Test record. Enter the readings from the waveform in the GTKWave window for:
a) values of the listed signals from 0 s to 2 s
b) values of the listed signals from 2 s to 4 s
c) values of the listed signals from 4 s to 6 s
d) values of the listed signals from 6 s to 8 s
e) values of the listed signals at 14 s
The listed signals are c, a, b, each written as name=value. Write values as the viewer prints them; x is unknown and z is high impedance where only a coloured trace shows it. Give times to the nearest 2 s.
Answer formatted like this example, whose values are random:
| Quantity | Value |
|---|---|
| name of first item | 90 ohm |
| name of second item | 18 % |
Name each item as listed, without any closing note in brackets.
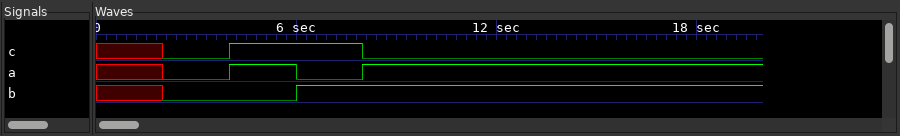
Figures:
| Quantity | Value |
|---|---|
| values of the listed signals from 0 s to 2 s | c=x, a=x, b=x |
| values of the listed signals from 2 s to 4 s | c=0, a=0, b=0 |
| values of the listed signals from 4 s to 6 s | c=1, a=1, b=0 |
| values of the listed signals from 6 s to 8 s | c=1, a=0, b=1 |
| values of the listed signals at 14 s | c=0, a=1, b=1 |
